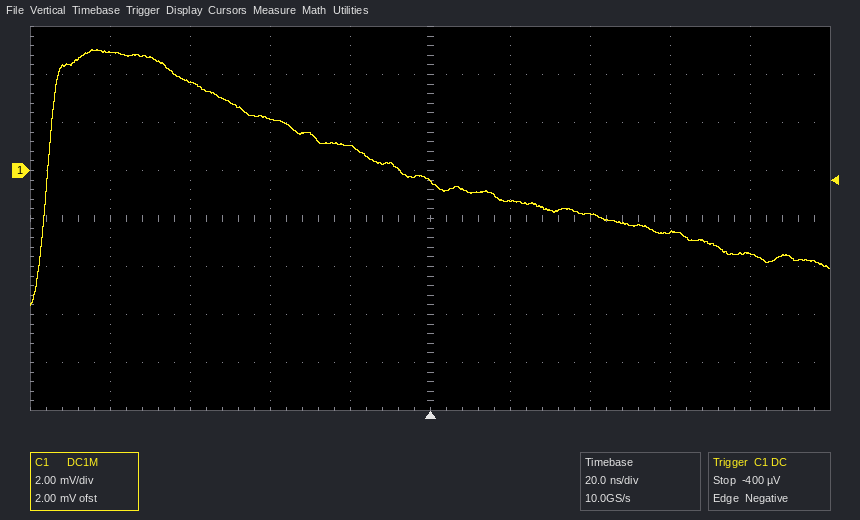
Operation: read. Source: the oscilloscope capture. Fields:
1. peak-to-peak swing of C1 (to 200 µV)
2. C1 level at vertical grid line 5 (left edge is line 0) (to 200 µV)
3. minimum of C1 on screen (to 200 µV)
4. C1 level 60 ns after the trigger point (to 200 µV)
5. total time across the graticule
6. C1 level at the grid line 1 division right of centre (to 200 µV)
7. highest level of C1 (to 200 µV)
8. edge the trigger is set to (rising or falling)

10.6 mV
-400 µV
-5.6 mV
-2.6 mV
200 ns
-1.2 mV
5.0 mV
falling
